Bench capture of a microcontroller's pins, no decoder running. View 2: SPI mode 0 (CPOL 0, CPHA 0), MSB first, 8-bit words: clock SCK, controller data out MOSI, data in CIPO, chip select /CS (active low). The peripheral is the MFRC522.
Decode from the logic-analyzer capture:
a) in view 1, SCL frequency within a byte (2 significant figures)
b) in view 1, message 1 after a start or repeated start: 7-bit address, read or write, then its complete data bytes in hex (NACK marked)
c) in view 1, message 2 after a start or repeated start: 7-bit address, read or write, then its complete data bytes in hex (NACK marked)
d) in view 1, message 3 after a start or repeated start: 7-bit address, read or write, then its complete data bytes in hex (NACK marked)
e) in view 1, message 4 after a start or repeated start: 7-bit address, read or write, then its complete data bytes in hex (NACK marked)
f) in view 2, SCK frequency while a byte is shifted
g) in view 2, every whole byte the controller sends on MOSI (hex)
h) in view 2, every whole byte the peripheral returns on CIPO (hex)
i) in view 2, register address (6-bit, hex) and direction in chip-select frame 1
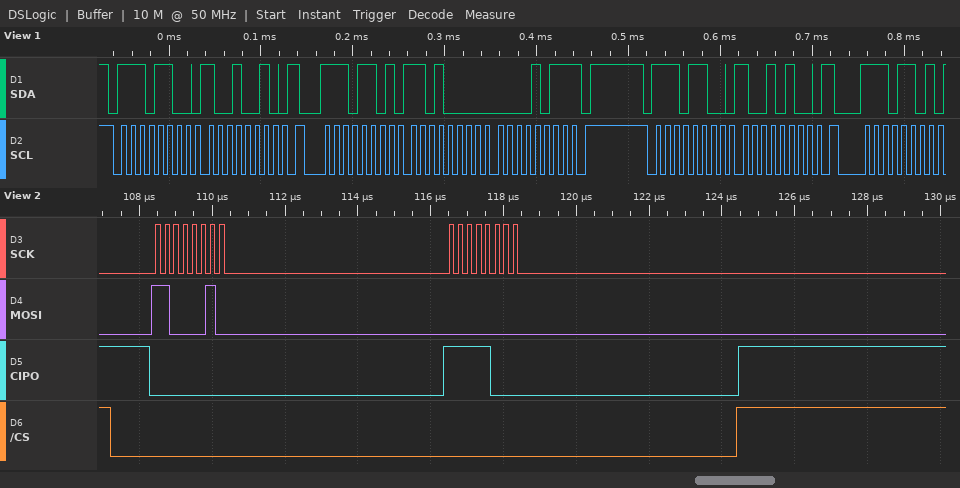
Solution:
100 kHz
0x76 write: 92
0x76 read: D0 0B NACK
0x76 write: 94
0x76 read
4 MHz
C2 00
00 F8
0x21 read
